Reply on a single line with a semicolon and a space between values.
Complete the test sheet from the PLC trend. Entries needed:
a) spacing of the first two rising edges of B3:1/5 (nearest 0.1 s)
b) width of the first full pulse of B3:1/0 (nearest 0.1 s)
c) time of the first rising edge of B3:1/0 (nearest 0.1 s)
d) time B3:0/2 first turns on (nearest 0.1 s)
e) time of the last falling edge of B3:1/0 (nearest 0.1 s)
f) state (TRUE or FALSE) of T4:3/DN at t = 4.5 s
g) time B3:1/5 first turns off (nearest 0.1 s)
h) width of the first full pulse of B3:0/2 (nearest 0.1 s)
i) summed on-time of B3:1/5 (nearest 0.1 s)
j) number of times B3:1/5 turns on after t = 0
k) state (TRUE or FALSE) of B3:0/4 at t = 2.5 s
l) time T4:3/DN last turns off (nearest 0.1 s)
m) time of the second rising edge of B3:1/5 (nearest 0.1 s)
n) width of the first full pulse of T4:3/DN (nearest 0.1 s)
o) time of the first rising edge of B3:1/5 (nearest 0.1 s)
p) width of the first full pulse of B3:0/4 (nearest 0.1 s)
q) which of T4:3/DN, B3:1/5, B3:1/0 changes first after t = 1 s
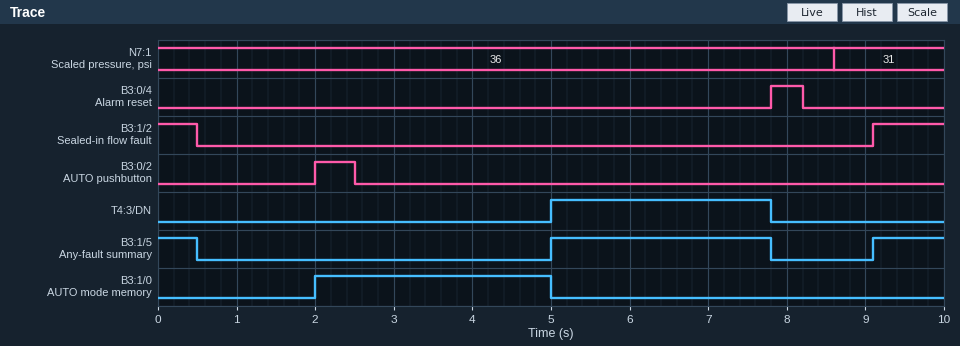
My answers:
4.1 s; 3.0 s; 2.0 s; 2.0 s; 5.0 s; FALSE; 0.5 s; 0.5 s; 4.2 s; 2; FALSE; 7.8 s; 9.1 s; 2.8 s; 5.0 s; 0.4 s; B3:1/0
